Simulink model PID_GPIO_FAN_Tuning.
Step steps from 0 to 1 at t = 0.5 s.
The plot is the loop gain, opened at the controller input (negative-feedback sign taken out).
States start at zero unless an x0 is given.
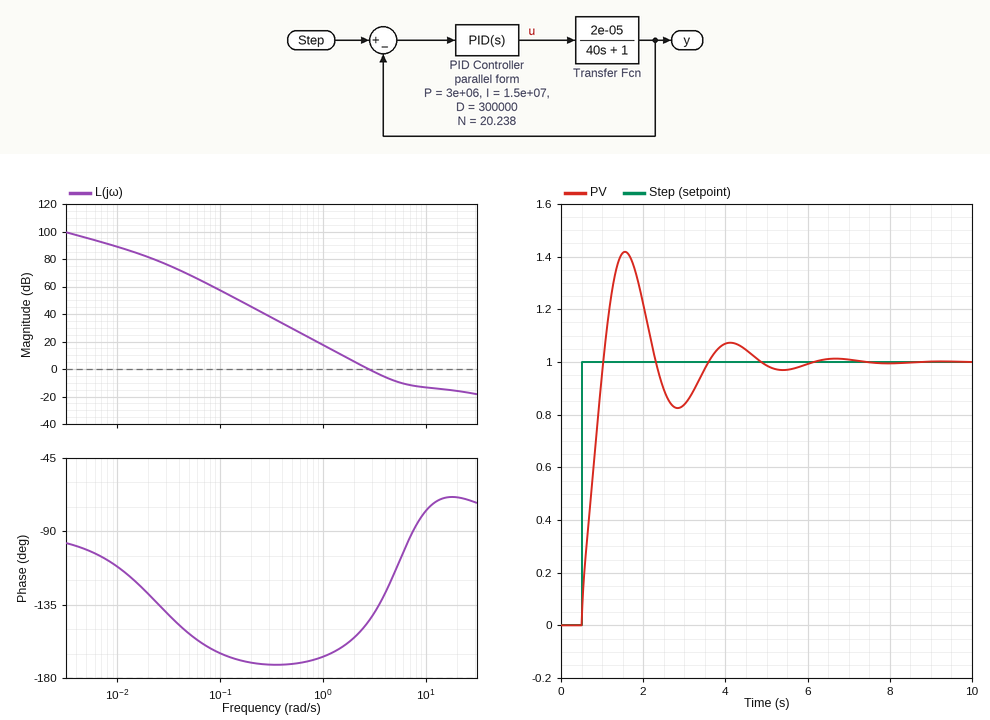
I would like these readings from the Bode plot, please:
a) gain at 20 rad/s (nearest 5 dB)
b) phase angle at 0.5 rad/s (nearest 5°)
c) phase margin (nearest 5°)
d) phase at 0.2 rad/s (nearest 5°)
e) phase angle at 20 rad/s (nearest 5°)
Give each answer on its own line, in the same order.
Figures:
-15 dB
-170°
35°
-170°
-70°
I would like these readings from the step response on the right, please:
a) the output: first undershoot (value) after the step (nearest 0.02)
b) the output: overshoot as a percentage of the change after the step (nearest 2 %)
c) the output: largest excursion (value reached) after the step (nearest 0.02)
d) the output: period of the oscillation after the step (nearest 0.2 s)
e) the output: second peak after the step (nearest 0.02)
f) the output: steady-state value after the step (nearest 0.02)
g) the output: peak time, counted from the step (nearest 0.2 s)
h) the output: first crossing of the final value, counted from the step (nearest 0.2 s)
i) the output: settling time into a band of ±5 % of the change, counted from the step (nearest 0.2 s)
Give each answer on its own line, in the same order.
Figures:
0.82
42 %
1.42
2.6 s
1.08
1.00
1.0 s
0.6 s
4.0 s
